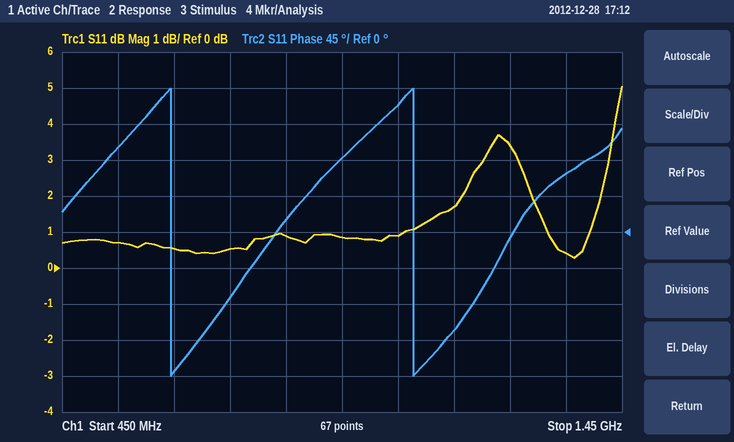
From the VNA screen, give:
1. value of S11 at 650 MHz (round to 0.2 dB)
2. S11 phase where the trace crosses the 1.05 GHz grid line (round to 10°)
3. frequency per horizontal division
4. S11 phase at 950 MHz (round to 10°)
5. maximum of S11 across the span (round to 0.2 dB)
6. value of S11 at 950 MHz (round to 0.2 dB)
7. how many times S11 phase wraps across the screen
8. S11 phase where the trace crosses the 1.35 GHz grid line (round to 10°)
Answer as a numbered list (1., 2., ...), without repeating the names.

1. 0.6 dB
2. 160°
3. 100 MHz
4. 90°
5. 5.0 dB
6. 0.8 dB
7. 2
8. 70°
